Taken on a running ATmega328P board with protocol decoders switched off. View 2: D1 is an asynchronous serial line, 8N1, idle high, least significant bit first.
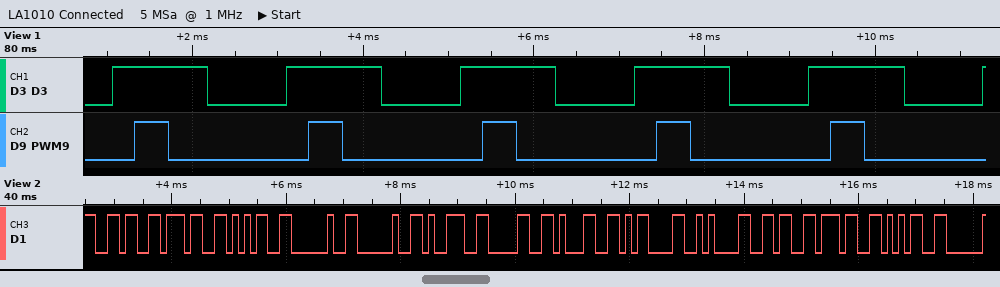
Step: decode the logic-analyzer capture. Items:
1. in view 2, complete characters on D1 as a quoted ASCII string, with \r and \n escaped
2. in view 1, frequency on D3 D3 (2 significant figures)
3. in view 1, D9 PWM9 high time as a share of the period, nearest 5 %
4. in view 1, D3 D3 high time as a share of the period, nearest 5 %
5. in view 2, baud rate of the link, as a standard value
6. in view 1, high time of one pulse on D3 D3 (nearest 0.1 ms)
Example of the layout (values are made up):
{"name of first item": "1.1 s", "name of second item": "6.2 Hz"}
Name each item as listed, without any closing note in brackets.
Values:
{"in view 2, complete characters on D1 as a quoted ASCII string, with \\r and \\n escaped": "\"675  901\\r\\n675\"", "in view 1, frequency on D3 D3": "490 Hz", "in view 1, D9 PWM9 high time as a share of the period, nearest 5 %": "20 %", "in view 1, D3 D3 high time as a share of the period, nearest 5 %": "55 %", "in view 2, baud rate of the link, as a standard value": "9600 baud", "in view 1, high time of one pulse on D3 D3": "1.1 ms"}
